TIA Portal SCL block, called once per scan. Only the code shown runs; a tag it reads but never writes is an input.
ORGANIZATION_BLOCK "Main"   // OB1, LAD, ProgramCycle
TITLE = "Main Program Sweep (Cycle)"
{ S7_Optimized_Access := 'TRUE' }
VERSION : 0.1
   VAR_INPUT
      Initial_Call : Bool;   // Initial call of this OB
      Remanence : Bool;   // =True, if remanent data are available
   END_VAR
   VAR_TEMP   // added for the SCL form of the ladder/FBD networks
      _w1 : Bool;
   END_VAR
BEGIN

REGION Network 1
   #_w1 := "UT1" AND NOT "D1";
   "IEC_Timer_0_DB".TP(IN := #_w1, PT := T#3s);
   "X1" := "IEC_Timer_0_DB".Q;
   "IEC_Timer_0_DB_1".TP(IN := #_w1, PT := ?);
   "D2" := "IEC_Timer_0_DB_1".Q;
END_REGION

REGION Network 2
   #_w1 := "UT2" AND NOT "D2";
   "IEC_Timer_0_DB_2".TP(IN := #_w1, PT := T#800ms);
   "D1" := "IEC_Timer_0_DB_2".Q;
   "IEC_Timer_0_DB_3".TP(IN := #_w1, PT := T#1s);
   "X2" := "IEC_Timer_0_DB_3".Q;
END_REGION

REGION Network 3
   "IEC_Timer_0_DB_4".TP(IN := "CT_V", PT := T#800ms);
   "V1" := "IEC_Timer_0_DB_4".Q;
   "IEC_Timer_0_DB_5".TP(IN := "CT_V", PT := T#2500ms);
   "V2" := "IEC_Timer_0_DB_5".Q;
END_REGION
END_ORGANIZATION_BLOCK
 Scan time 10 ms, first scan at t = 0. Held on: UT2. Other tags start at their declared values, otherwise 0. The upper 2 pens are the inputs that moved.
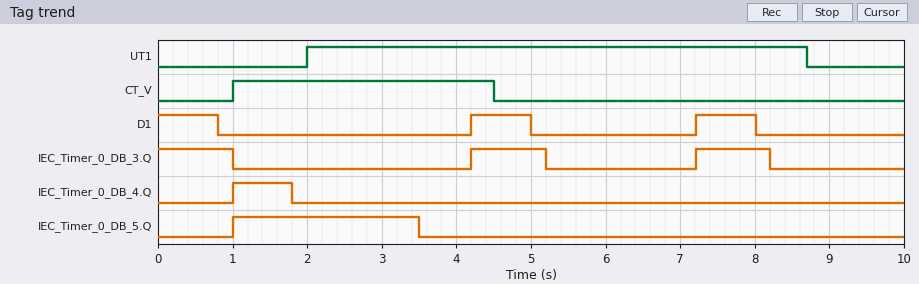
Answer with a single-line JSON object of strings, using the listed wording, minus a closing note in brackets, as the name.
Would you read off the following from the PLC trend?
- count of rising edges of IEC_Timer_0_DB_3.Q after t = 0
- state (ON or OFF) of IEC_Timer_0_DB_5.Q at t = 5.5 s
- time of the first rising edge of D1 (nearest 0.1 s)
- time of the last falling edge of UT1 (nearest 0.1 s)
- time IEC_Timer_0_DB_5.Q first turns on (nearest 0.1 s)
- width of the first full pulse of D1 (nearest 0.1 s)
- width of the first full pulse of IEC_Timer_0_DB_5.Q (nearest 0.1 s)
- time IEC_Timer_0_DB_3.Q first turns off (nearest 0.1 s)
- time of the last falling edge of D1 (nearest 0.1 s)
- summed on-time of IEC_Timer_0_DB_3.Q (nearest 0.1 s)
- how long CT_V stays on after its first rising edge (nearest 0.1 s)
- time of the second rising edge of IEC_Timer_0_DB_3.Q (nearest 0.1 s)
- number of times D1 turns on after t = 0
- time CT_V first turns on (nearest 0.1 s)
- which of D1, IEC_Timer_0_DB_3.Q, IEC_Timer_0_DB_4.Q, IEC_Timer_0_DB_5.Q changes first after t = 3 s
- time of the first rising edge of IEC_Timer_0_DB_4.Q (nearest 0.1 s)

{"count of rising edges of IEC_Timer_0_DB_3.Q after t = 0": "2", "state (ON or OFF) of IEC_Timer_0_DB_5.Q at t = 5.5 s": "OFF", "time of the first rising edge of D1": "4.2 s", "time of the last falling edge of UT1": "8.7 s", "time IEC_Timer_0_DB_5.Q first turns on": "1.0 s", "width of the first full pulse of D1": "0.8 s", "width of the first full pulse of IEC_Timer_0_DB_5.Q": "2.5 s", "time IEC_Timer_0_DB_3.Q first turns off": "1.0 s", "time of the last falling edge of D1": "8.0 s", "summed on-time of IEC_Timer_0_DB_3.Q": "3.0 s", "how long CT_V stays on after its first rising edge": "3.5 s", "time of the second rising edge of IEC_Timer_0_DB_3.Q": "7.2 s", "number of times D1 turns on after t = 0": "2", "time CT_V first turns on": "1.0 s", "which of D1, IEC_Timer_0_DB_3.Q, IEC_Timer_0_DB_4.Q, IEC_Timer_0_DB_5.Q changes first after t = 3 s": "IEC_Timer_0_DB_5.Q", "time of the first rising edge of IEC_Timer_0_DB_4.Q": "1.0 s"}
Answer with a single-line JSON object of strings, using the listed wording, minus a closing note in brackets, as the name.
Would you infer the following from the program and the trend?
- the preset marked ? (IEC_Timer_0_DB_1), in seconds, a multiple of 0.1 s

{"the preset marked ? (IEC_Timer_0_DB_1), in seconds, a multiple of 0.1 s": "2.2 s"}
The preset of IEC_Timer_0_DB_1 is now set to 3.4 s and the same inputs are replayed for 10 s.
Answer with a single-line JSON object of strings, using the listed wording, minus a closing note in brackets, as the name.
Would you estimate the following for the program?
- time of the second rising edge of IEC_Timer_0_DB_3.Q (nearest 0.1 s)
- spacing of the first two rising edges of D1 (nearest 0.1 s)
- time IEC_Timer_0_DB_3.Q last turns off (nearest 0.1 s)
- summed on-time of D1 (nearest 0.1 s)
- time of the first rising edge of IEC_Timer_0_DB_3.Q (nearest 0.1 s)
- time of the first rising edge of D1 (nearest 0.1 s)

{"time of the second rising edge of IEC_Timer_0_DB_3.Q": "9.6 s", "spacing of the first two rising edges of D1": "4.2 s", "time IEC_Timer_0_DB_3.Q last turns off": "6.4 s", "summed on-time of D1": "2.0 s", "time of the first rising edge of IEC_Timer_0_DB_3.Q": "5.4 s", "time of the first rising edge of D1": "5.4 s"}
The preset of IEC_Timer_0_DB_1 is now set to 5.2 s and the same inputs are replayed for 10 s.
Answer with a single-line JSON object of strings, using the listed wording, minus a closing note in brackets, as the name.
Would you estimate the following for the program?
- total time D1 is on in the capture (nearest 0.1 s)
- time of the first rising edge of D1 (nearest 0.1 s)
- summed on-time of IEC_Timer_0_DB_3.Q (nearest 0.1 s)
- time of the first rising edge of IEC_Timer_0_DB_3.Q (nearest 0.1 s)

{"total time D1 is on in the capture": "1.6 s", "time of the first rising edge of D1": "7.2 s", "summed on-time of IEC_Timer_0_DB_3.Q": "2.0 s", "time of the first rising edge of IEC_Timer_0_DB_3.Q": "7.2 s"}
